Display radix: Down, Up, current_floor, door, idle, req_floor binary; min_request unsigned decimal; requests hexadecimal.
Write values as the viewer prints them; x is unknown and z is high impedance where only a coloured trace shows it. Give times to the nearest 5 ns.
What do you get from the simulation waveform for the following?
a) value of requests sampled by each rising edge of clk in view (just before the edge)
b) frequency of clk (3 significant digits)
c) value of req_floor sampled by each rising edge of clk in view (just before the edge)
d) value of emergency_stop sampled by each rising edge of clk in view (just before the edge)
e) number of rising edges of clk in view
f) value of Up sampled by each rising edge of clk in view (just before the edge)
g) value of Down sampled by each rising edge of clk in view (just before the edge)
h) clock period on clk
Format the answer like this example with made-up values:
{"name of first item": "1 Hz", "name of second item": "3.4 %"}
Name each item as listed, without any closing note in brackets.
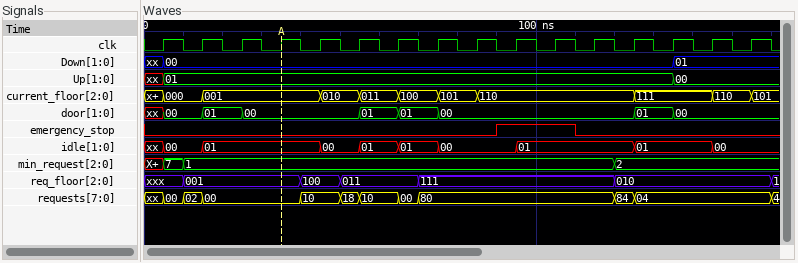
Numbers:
{"value of requests sampled by each rising edge of clk in view": "xx, 02, 00, 00, 10, 18, 10, 80, 80, 80, 80, 80, 84, 04, 04, 04", "frequency of clk": "100 MHz", "value of req_floor sampled by each rising edge of clk in view": "xxx, 001, 001, 001, 100, 011, 011, 111, 111, 111, 111, 111, 010, 010, 010, 010", "value of emergency_stop sampled by each rising edge of clk in view": "0 0 0 0 0 0 0 0 0 1 1 0 0 0 0 0", "number of rising edges of clk in view": "16", "value of Up sampled by each rising edge of clk in view": "xx, 01, 01, 01, 01, 01, 01, 01, 01, 01, 01, 01, 01, 01, 00, 00", "value of Down sampled by each rising edge of clk in view": "xx, 00, 00, 00, 00, 00, 00, 00, 00, 00, 00, 00, 00, 00, 01, 01", "clock period on clk": "10 ns"}
